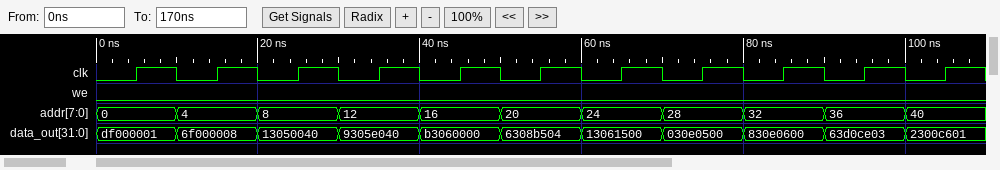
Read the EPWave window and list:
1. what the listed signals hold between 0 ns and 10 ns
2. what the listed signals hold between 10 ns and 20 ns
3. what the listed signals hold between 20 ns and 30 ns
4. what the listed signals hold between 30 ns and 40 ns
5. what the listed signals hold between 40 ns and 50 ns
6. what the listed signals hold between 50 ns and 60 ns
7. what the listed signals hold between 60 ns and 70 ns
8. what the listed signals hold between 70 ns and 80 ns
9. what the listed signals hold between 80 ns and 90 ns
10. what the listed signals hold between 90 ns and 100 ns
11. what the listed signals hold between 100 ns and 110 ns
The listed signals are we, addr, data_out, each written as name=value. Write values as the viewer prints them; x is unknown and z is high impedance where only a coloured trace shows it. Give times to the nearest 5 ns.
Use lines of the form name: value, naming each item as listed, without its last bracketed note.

what the listed signals hold between 0 ns and 10 ns: we=0, addr=0, data_out=df000001
what the listed signals hold between 10 ns and 20 ns: we=0, addr=4, data_out=6f000008
what the listed signals hold between 20 ns and 30 ns: we=0, addr=8, data_out=13050040
what the listed signals hold between 30 ns and 40 ns: we=0, addr=12, data_out=9305e040
what the listed signals hold between 40 ns and 50 ns: we=0, addr=16, data_out=b3060000
what the listed signals hold between 50 ns and 60 ns: we=0, addr=20, data_out=6308b504
what the listed signals hold between 60 ns and 70 ns: we=0, addr=24, data_out=13061500
what the listed signals hold between 70 ns and 80 ns: we=0, addr=28, data_out=030e0500
what the listed signals hold between 80 ns and 90 ns: we=0, addr=32, data_out=830e0600
what the listed signals hold between 90 ns and 100 ns: we=0, addr=36, data_out=63d0ce03
what the listed signals hold between 100 ns and 110 ns: we=0, addr=40, data_out=2300c601
